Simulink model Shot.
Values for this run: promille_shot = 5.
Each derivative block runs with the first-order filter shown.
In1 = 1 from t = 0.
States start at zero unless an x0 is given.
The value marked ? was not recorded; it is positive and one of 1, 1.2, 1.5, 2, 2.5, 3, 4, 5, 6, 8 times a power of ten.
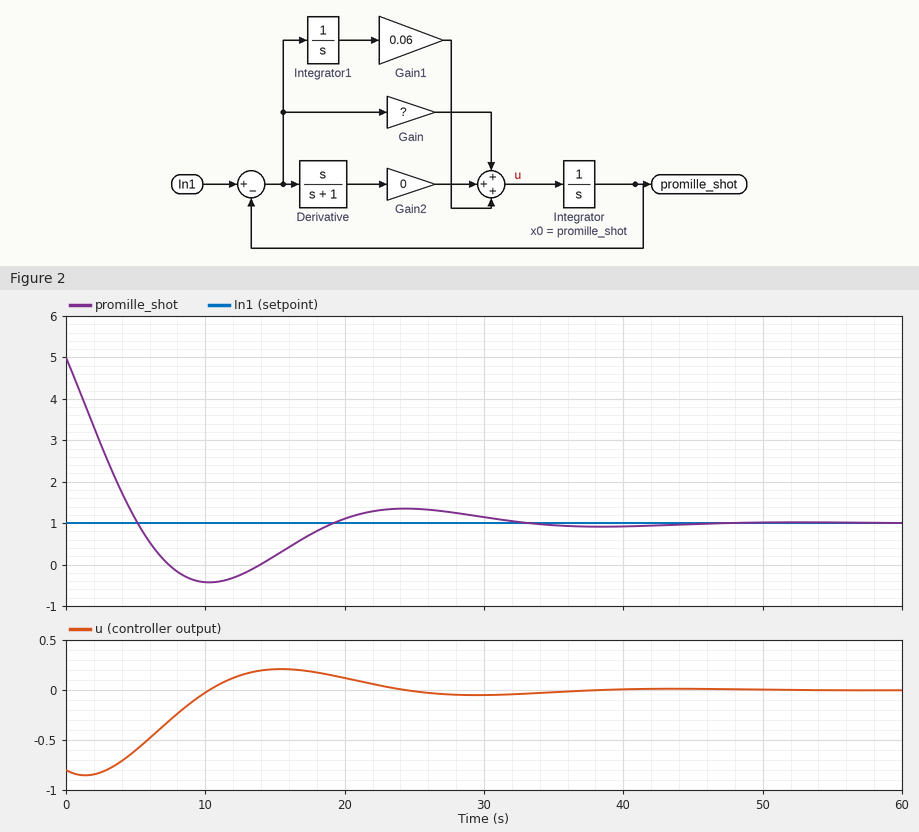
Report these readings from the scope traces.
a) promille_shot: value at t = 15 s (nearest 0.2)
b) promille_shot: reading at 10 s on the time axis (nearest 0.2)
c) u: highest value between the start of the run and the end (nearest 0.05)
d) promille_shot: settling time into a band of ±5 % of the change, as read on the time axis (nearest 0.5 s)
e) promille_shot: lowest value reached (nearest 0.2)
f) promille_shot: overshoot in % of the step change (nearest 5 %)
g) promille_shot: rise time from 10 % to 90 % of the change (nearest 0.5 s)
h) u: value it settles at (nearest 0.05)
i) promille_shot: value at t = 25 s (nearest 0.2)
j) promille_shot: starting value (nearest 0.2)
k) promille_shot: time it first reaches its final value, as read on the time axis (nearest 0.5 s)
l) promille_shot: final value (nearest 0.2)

0.2
-0.4
0.20
29.0 s
-0.4
35 %
4.0 s
0.00
1.4
5.0
5.0 s
1.0
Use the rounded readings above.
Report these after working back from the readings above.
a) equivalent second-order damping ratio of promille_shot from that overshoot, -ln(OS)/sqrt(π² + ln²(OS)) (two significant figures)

0.32
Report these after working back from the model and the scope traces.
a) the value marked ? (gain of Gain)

0.2
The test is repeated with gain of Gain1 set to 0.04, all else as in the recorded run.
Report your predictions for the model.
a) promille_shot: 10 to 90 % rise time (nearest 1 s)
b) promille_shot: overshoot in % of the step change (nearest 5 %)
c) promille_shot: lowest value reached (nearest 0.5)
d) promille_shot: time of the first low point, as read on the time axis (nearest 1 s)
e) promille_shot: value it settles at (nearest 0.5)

5 s
30 %
0.0
12 s
1.0
